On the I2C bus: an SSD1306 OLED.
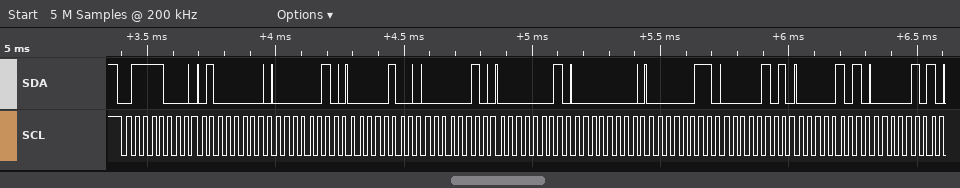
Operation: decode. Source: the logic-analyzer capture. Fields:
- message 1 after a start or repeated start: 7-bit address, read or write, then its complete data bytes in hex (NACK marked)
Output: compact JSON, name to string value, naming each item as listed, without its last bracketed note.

{"message 1 after a start or repeated start: 7-bit address, read or write, then its complete data bytes in hex": "0x3C write: 40 02 04 02 01 00 03 05 05 05"}
